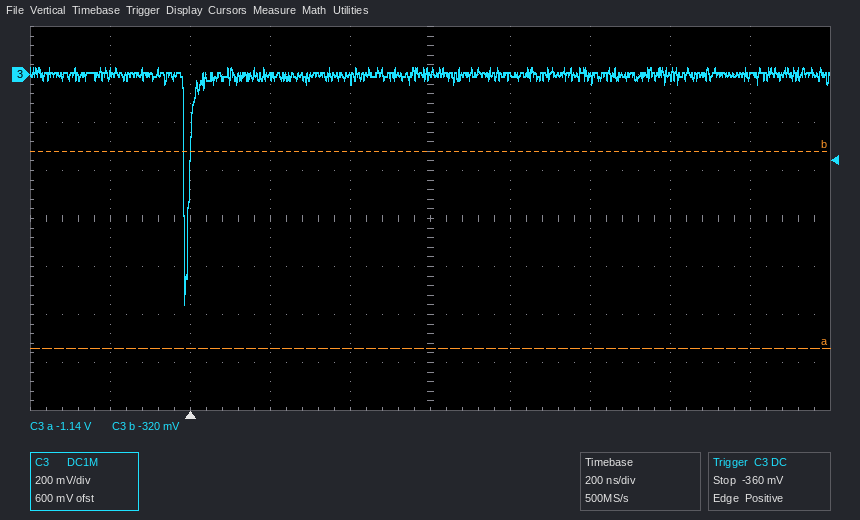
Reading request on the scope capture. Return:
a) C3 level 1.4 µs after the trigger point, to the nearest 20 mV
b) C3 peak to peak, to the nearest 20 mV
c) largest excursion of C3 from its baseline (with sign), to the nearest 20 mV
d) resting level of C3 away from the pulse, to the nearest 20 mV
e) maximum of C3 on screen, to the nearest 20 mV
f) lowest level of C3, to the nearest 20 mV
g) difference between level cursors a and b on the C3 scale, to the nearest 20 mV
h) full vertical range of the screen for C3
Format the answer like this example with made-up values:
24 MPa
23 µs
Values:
0 mV
980 mV
-960 mV
0 mV
20 mV
-960 mV
820 mV
1.6 V
